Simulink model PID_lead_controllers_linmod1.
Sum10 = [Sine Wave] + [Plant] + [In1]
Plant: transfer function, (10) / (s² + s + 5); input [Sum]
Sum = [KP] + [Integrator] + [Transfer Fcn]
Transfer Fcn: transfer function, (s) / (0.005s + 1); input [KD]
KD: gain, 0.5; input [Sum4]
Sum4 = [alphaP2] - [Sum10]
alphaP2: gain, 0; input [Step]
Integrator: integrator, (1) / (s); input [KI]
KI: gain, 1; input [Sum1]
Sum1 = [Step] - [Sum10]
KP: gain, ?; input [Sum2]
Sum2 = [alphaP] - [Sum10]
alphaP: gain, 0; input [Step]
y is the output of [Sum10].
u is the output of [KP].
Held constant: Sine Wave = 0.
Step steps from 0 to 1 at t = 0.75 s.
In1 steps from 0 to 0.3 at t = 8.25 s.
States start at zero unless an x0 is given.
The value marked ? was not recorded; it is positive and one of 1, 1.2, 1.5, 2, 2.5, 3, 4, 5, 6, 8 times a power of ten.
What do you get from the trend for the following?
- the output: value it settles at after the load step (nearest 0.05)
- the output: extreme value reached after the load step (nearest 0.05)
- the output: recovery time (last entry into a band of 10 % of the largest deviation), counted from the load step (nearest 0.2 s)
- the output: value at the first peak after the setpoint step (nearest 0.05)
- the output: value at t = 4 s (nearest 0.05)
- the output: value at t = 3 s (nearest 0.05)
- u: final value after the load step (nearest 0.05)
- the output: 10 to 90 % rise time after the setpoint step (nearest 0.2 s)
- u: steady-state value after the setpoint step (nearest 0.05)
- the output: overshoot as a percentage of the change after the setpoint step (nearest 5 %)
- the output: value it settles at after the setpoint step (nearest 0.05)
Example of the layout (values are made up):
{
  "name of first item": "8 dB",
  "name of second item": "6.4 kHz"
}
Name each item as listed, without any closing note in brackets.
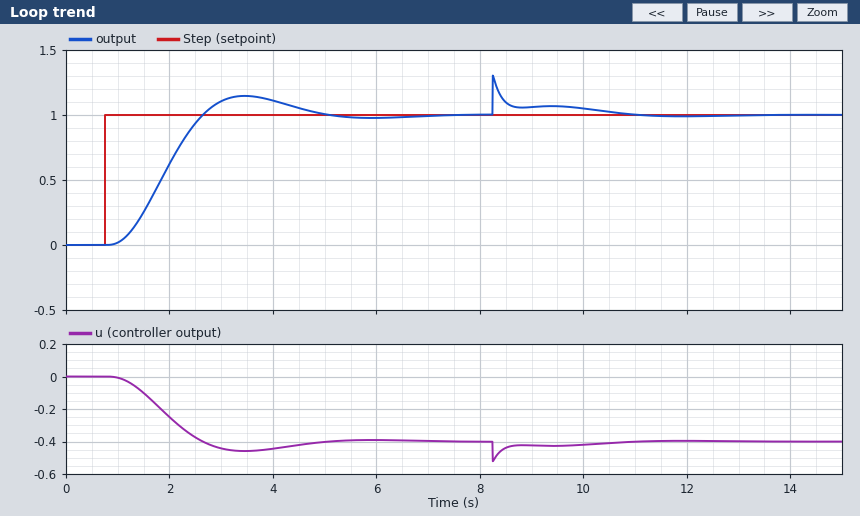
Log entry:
{
  "the output: value it settles at after the load step": "1.00",
  "the output: extreme value reached after the load step": "1.30",
  "the output: recovery time (last entry into a band of 10 % of the largest deviation), counted from the load step": "2.2 s",
  "the output: value at the first peak after the setpoint step": "1.15",
  "the output: value at t = 4 s": "1.10",
  "the output: value at t = 3 s": "1.10",
  "u: final value after the load step": "-0.40",
  "the output: 10 to 90 % rise time after the setpoint step": "1.2 s",
  "u: steady-state value after the setpoint step": "-0.40",
  "the output: overshoot as a percentage of the change after the setpoint step": "15 %",
  "the output: value it settles at after the setpoint step": "1.00"
}
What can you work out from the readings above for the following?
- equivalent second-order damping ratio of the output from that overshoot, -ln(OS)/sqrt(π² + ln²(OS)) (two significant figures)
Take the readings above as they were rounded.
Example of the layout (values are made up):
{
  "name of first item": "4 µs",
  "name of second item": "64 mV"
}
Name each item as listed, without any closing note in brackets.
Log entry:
{
  "equivalent second-order damping ratio of the output from that overshoot, -ln(OS)/sqrt(π² + ln²(OS))": "0.52"
}
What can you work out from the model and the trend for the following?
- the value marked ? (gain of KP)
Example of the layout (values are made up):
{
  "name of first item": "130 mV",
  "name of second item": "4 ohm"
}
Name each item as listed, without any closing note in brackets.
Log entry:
{
  "the value marked ?": "0.4"
}
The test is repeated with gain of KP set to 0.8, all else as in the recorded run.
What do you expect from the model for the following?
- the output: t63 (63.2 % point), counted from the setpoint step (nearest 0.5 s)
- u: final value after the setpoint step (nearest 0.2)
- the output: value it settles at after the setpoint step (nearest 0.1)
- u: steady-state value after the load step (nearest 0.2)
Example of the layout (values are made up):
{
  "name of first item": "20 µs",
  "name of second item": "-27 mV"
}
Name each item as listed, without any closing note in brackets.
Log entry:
{
  "the output: t63 (63.2 % point), counted from the setpoint step": "1.5 s",
  "u: final value after the setpoint step": "-0.8",
  "the output: value it settles at after the setpoint step": "1.0",
  "u: steady-state value after the load step": "-0.8"
}
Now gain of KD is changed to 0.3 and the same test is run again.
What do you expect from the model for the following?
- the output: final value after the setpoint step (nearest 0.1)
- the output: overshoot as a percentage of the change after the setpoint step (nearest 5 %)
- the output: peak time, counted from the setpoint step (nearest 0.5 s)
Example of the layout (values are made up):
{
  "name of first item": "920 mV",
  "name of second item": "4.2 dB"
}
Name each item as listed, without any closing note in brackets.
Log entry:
{
  "the output: final value after the setpoint step": "1.0",
  "the output: overshoot as a percentage of the change after the setpoint step": "10 %",
  "the output: peak time, counted from the setpoint step": "2.0 s"
}
